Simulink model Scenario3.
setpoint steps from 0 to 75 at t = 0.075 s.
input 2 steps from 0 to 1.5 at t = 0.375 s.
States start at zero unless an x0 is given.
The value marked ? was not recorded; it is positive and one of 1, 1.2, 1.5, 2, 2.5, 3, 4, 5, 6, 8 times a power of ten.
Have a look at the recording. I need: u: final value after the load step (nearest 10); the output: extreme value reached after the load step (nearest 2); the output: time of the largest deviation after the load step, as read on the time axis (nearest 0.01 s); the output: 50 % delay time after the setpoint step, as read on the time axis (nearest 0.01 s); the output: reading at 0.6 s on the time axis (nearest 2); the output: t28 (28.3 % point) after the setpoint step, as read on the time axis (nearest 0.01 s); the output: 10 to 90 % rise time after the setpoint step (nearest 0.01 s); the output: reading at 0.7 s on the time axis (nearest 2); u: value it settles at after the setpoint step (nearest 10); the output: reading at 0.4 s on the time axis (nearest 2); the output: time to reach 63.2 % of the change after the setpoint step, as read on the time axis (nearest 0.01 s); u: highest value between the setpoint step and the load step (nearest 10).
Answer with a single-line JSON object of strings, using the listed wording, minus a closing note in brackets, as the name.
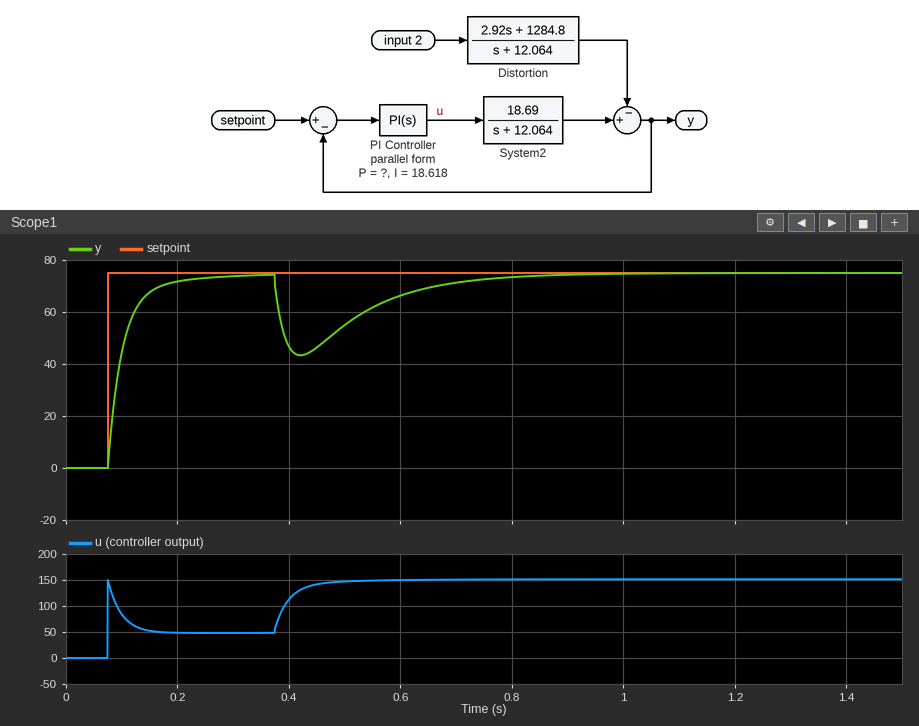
{"u: final value after the load step": "150", "the output: extreme value reached after the load step": "44", "the output: time of the largest deviation after the load step, as read on the time axis": "0.42 s", "the output: 50 % delay time after the setpoint step, as read on the time axis": "0.09 s", "the output: reading at 0.6 s on the time axis": "66", "the output: t28 (28.3 % point) after the setpoint step, as read on the time axis": "0.08 s", "the output: 10 to 90 % rise time after the setpoint step": "0.07 s", "the output: reading at 0.7 s on the time axis": "72", "u: value it settles at after the setpoint step": "50", "the output: reading at 0.4 s on the time axis": "46", "the output: time to reach 63.2 % of the change after the setpoint step, as read on the time axis": "0.10 s", "u: highest value between the setpoint step and the load step": "150"}
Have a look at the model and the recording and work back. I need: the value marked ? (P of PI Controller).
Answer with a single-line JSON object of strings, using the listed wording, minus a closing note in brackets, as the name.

{"the value marked ?": "2"}
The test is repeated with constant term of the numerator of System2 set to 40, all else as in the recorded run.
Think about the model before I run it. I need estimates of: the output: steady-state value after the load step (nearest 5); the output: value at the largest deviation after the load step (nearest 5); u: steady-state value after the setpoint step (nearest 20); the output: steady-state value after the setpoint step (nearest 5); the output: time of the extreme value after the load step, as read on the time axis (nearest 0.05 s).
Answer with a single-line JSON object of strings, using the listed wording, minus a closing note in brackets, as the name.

{"the output: steady-state value after the load step": "75", "the output: value at the largest deviation after the load step": "55", "u: steady-state value after the setpoint step": "20", "the output: steady-state value after the setpoint step": "75", "the output: time of the extreme value after the load step, as read on the time axis": "0.40 s"}
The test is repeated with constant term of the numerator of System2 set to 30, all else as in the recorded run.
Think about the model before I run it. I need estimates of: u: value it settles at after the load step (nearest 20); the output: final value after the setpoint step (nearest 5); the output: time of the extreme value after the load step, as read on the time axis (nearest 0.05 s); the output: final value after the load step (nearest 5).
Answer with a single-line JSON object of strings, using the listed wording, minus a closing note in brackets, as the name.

{"u: value it settles at after the load step": "100", "the output: final value after the setpoint step": "75", "the output: time of the extreme value after the load step, as read on the time axis": "0.40 s", "the output: final value after the load step": "75"}
